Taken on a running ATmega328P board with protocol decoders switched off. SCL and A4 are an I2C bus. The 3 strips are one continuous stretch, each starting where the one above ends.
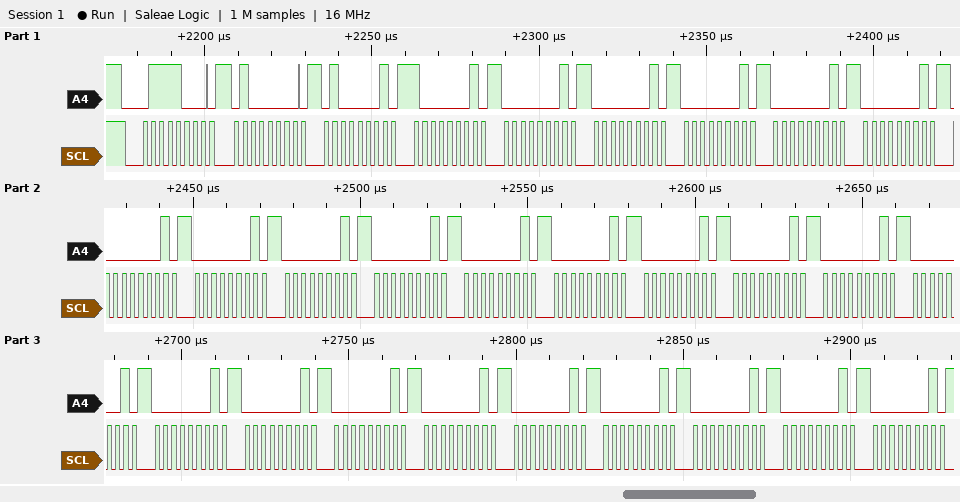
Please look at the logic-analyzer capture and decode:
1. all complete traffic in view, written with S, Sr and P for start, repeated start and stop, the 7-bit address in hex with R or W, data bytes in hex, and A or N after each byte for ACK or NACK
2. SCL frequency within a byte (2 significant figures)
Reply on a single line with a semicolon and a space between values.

S 3CW A 40 A 41 A 81 A 01 A 01 A 01 A 01 A 01 A 01 A 01 A 01 A 01 A 01 A 01 A 01 A 01 A 01 A 01 A 01 A 01 A 01 A 01 A 01 A 01 A 01 A 01 A 01 A; 400 kHz
